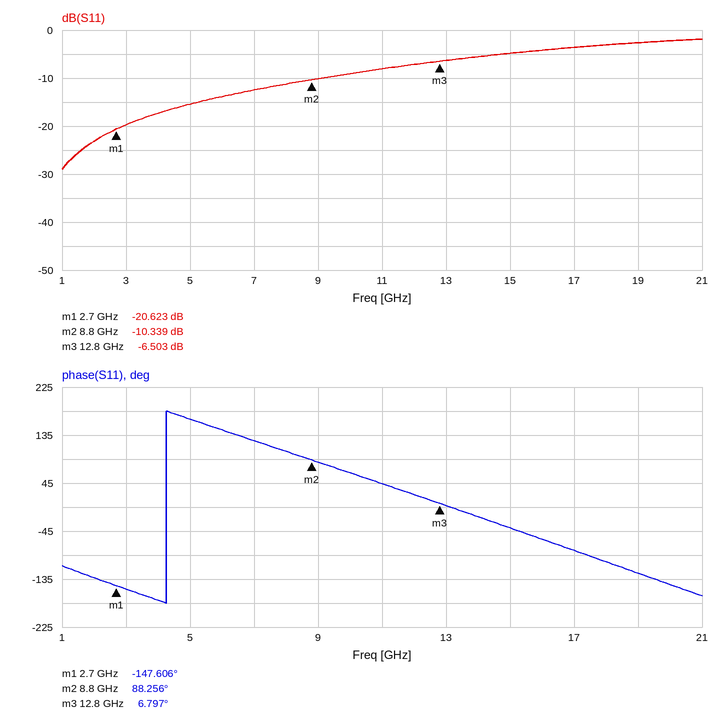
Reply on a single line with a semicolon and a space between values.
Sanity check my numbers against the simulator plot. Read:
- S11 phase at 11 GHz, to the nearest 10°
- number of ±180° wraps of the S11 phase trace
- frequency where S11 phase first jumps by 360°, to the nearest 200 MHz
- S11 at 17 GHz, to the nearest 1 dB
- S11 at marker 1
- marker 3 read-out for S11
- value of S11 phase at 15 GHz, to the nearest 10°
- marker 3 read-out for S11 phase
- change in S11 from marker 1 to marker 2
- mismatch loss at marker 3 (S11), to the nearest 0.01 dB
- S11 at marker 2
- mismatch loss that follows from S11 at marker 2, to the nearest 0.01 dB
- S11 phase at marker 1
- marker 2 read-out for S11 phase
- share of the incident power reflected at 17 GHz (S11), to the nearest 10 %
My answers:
40°; 1; 4.2 GHz; -4 dB; -20.623 dB; -6.503 dB; -40°; 6.797°; 10.284 dB; 1.10 dB; -10.339 dB; 0.42 dB; -147.606°; 88.256°; 40 %
